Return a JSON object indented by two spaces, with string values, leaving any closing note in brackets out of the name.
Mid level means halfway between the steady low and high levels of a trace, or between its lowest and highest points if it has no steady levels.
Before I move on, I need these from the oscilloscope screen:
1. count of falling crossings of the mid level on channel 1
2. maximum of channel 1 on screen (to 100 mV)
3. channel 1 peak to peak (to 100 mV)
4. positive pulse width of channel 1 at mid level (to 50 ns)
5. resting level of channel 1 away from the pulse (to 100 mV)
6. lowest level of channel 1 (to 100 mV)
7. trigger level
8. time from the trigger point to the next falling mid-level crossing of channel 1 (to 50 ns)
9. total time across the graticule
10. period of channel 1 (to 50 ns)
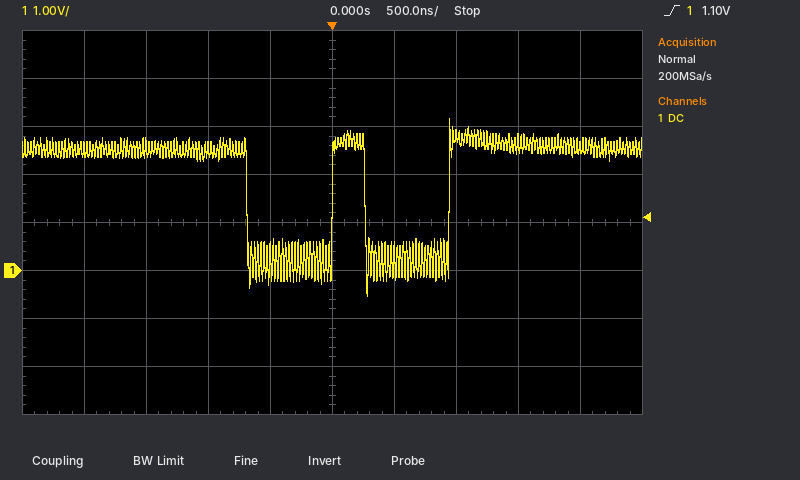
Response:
{
  "count of falling crossings of the mid level on channel 1": "2",
  "maximum of channel 1 on screen": "3.2 V",
  "channel 1 peak to peak": "3.7 V",
  "positive pulse width of channel 1 at mid level": "250 ns",
  "resting level of channel 1 away from the pulse": "2.5 V",
  "lowest level of channel 1": "-500 mV",
  "trigger level": "1.10 V",
  "time from the trigger point to the next falling mid-level crossing of channel 1": "250 ns",
  "total time across the graticule": "5 µs",
  "period of channel 1": "950 ns"
}
